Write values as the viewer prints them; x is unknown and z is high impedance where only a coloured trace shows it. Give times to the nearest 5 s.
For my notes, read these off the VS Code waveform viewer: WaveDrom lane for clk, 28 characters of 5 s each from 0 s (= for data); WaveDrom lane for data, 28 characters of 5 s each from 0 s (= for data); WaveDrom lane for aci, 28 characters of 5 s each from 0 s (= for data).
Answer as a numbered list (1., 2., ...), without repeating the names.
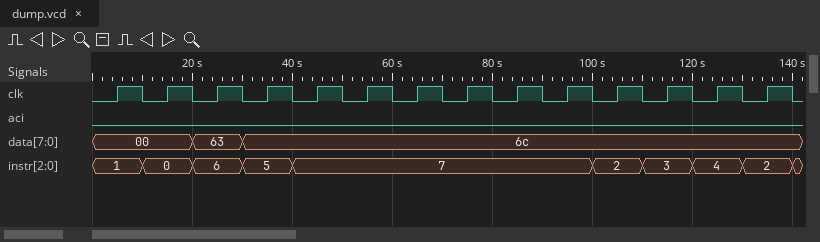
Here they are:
1. {name: 'clk', wave: '0101010101010101010101010101'}
2. {name: 'data', wave: '=...=.=.....................', data: '00 63 6c'}
3. {name: 'aci', wave: '0...........................'}
